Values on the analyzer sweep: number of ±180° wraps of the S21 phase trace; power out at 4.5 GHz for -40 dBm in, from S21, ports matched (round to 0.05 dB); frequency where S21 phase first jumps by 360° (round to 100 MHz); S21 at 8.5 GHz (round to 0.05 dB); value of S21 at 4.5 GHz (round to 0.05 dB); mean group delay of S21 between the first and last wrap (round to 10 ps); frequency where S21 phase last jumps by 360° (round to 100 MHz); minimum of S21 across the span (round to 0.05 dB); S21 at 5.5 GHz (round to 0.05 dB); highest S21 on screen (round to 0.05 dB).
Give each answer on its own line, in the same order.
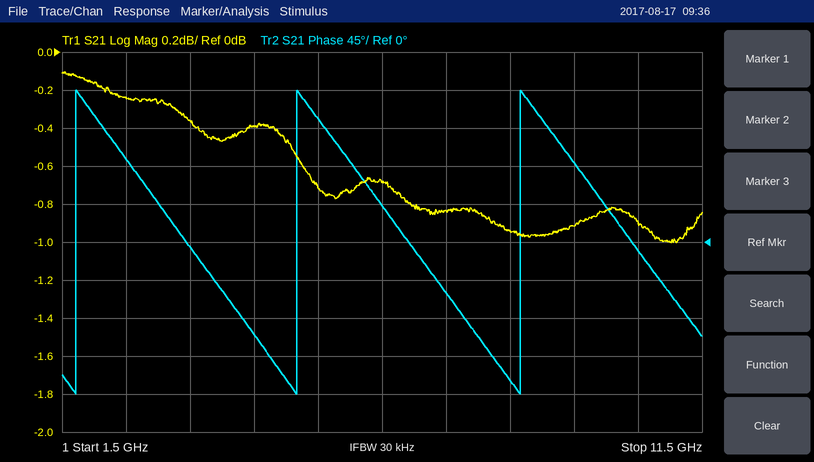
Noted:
3
-40.40 dBm
1.7 GHz
-0.95 dB
-0.40 dB
290 ps
8.7 GHz
-1.00 dB
-0.70 dB
-0.10 dB
